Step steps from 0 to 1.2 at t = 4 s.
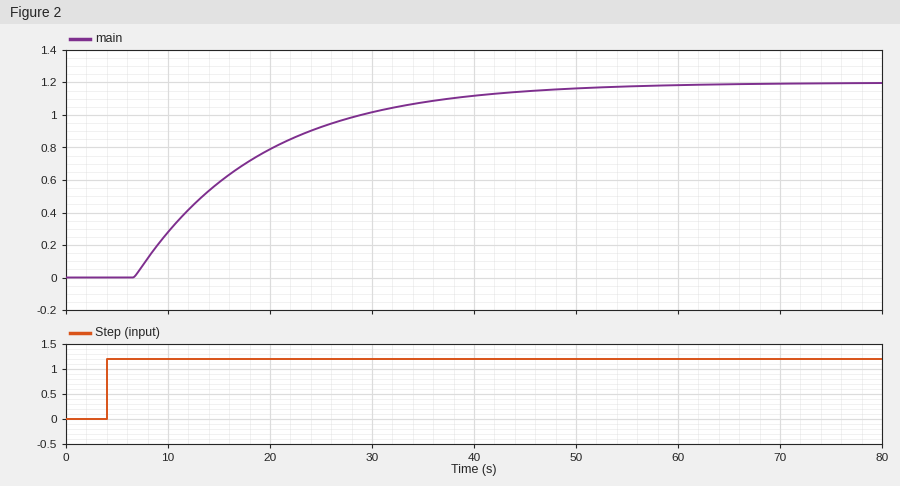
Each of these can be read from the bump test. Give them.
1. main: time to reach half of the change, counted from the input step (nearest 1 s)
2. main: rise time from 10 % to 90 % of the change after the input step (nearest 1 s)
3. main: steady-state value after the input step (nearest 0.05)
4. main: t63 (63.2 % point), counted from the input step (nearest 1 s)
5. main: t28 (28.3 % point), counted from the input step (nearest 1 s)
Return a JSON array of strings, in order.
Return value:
["11 s", "27 s", "1.20", "15 s", "7 s"]
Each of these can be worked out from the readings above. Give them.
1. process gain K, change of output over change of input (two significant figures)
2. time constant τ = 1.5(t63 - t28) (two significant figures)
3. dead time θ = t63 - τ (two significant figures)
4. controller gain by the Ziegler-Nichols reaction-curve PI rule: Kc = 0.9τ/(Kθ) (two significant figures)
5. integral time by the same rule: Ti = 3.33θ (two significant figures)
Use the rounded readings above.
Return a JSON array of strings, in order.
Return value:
["1.0", "12 s", "3.0 s", "3.6", "10.0 s"]
